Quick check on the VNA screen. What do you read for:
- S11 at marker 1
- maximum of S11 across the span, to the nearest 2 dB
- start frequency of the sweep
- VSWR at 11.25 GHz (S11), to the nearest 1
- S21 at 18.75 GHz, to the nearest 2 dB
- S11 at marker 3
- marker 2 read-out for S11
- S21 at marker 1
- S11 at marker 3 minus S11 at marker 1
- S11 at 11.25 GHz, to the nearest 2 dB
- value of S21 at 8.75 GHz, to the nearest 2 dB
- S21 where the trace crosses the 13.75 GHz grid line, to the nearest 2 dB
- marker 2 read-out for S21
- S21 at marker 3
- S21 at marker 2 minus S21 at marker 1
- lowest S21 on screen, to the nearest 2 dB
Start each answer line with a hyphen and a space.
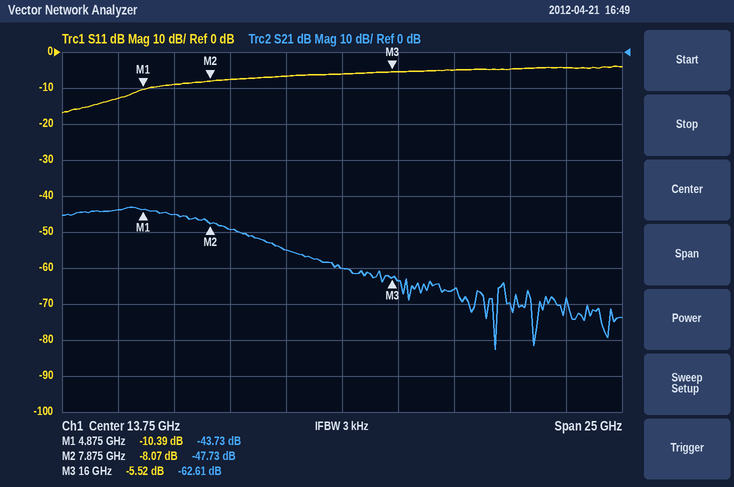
- -10.39 dB
- -4 dB
- 1.25 GHz
- 3
- -66 dB
- -5.52 dB
- -8.07 dB
- -43.73 dB
- 4.87 dB
- -6 dB
- -50 dB
- -60 dB
- -47.73 dB
- -62.61 dB
- -4.00 dB
- -82 dB
